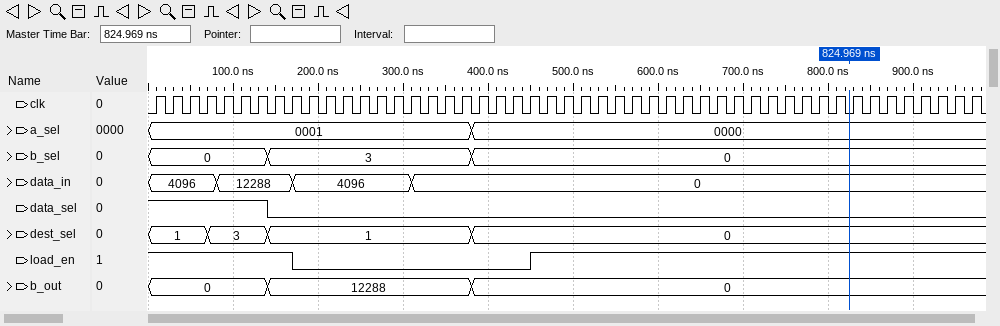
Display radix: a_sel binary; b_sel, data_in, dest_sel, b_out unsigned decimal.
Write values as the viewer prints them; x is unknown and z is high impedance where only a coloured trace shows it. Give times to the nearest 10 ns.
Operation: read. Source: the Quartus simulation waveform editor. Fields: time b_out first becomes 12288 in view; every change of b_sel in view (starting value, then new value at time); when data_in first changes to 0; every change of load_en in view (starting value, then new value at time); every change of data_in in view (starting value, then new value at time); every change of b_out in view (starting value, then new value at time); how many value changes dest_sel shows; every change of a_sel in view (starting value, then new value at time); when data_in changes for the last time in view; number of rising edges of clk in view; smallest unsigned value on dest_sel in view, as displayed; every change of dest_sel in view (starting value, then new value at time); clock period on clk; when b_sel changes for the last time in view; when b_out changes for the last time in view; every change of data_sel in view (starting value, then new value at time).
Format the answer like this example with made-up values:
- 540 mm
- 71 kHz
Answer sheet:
- 140 ns
- 0, 3 at 140 ns, 0 at 380 ns
- 310 ns
- 1, 0 at 170 ns, 1 at 450 ns
- 4096, 12288 at 80 ns, 4096 at 170 ns, 0 at 310 ns
- 0, 12288 at 140 ns, 0 at 380 ns
- 3
- 0001, 0000 at 380 ns
- 310 ns
- 49
- 0
- 1, 3 at 70 ns, 1 at 140 ns, 0 at 380 ns
- 20 ns
- 380 ns
- 380 ns
- 1, 0 at 140 ns
